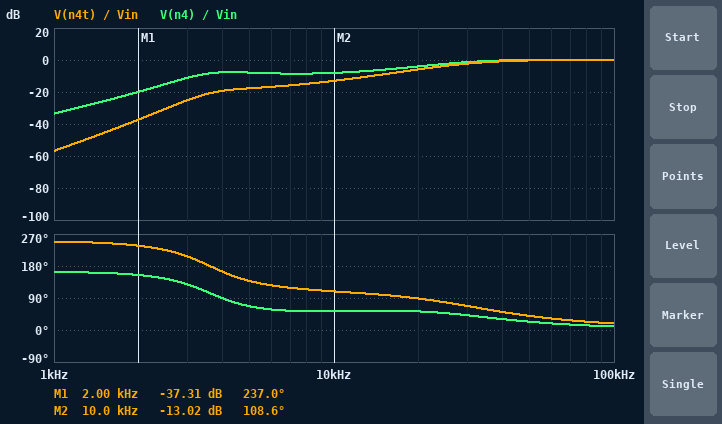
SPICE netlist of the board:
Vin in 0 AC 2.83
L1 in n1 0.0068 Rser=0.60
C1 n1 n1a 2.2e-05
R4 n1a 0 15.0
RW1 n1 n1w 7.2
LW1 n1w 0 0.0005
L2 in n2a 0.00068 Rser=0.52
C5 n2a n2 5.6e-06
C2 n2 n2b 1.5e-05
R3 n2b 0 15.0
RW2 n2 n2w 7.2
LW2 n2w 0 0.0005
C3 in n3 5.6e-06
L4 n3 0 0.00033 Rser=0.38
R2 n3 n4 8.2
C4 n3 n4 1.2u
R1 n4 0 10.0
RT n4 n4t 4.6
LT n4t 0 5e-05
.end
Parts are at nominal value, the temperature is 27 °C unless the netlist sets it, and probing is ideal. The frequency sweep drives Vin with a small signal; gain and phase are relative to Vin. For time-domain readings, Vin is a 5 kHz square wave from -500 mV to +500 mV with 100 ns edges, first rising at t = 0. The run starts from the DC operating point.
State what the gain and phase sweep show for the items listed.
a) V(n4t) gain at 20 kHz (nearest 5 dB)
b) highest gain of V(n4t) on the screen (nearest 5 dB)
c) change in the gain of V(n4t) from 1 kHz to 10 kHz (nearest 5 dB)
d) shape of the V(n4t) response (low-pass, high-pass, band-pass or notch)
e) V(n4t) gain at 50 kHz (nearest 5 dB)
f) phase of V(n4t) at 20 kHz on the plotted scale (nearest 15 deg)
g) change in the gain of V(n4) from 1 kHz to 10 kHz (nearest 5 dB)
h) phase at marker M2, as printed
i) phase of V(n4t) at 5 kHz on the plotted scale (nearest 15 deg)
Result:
-5 dB
0 dB
45 dB
high-pass
0 dB
90 deg
25 dB
108.6 deg
135 deg
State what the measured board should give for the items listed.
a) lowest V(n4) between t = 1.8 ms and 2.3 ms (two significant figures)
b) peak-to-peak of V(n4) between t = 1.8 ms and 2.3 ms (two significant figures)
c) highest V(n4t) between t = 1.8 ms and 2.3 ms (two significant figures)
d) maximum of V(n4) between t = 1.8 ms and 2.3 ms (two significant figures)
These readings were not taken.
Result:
-1.1 V
2.2 V
1.0 V
1.1 V
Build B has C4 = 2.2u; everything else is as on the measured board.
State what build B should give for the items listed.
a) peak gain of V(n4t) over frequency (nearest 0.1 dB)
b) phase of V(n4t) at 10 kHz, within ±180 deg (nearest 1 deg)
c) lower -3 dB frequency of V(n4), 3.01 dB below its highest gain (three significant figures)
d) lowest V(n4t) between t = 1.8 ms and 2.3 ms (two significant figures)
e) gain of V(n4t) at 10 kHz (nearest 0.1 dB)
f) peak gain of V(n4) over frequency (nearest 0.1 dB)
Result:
0.2 dB
118 deg
17.4 kHz
-1.0 V
-11.6 dB
0.6 dB
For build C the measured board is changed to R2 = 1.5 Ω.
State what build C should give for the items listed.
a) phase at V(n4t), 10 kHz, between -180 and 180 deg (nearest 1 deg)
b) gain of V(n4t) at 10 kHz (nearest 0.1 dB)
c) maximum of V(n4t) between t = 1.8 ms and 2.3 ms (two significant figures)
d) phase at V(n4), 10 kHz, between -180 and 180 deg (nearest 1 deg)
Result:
101 deg
-6.8 dB
990 mV
45 deg
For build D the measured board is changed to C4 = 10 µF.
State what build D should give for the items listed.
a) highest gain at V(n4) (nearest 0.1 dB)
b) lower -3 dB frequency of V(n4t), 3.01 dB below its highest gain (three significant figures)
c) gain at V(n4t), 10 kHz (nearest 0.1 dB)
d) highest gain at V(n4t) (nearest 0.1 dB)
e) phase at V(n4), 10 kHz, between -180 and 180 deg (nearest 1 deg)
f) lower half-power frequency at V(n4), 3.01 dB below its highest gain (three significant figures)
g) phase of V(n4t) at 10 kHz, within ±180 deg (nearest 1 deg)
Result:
1.4 dB
13.4 kHz
-6.4 dB
0.1 dB
65 deg
9.78 kHz
120 deg
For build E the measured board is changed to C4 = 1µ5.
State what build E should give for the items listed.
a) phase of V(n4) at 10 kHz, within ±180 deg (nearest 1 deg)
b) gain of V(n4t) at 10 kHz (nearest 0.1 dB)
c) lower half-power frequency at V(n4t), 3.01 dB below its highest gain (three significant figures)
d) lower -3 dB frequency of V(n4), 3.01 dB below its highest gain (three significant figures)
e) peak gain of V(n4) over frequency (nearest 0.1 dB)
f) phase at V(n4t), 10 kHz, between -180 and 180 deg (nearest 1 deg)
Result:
57 deg
-12.6 dB
24.4 kHz
20.9 kHz
0.3 dB
112 deg
